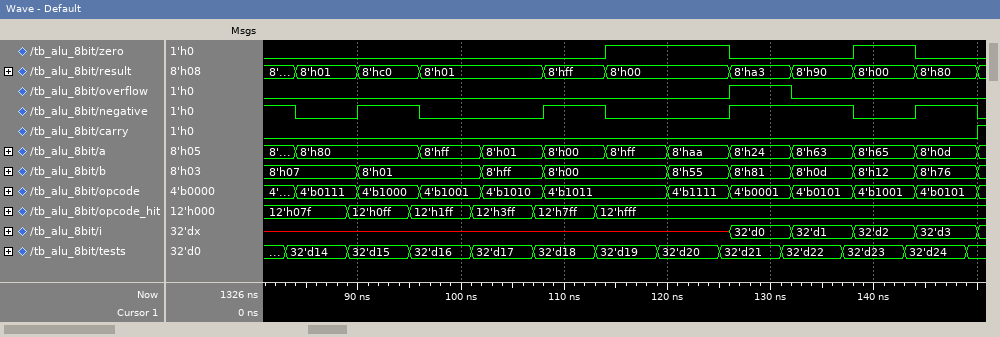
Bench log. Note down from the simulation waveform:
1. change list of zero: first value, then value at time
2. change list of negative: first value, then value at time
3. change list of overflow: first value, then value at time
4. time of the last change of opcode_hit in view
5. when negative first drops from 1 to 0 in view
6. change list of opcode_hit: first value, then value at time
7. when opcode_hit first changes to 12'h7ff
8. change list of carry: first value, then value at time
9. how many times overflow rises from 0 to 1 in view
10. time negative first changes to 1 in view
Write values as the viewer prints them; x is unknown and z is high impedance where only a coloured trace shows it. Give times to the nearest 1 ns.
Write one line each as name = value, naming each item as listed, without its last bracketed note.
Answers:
change list of zero: first value, then value at time = 0, 1 at 114 ns, 0 at 126 ns, 1 at 138 ns, 0 at 144 ns
change list of negative: first value, then value at time = 1, 0 at 84 ns, 1 at 90 ns, 0 at 96 ns, 1 at 108 ns, 0 at 114 ns, 1 at 126 ns, 0 at 138 ns, 1 at 144 ns, 0 at 150 ns
change list of overflow: first value, then value at time = 0, 1 at 126 ns, 0 at 132 ns
time of the last change of opcode_hit in view = 113 ns
when negative first drops from 1 to 0 in view = 84 ns
change list of opcode_hit: first value, then value at time = 12'h07f, 12'h0ff at 89 ns, 12'h1ff at 95 ns, 12'h3ff at 101 ns, 12'h7ff at 107 ns, 12'hfff at 113 ns
when opcode_hit first changes to 12'h7ff = 107 ns
change list of carry: first value, then value at time = 0, 1 at 150 ns
how many times overflow rises from 0 to 1 in view = 1
time negative first changes to 1 in view = 90 ns
